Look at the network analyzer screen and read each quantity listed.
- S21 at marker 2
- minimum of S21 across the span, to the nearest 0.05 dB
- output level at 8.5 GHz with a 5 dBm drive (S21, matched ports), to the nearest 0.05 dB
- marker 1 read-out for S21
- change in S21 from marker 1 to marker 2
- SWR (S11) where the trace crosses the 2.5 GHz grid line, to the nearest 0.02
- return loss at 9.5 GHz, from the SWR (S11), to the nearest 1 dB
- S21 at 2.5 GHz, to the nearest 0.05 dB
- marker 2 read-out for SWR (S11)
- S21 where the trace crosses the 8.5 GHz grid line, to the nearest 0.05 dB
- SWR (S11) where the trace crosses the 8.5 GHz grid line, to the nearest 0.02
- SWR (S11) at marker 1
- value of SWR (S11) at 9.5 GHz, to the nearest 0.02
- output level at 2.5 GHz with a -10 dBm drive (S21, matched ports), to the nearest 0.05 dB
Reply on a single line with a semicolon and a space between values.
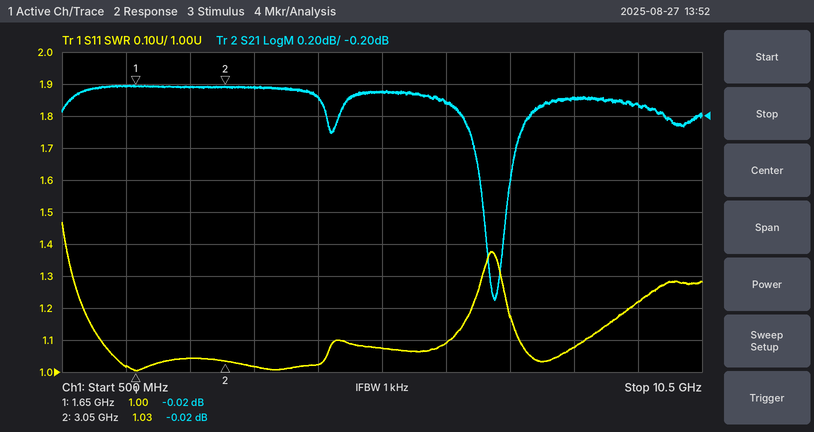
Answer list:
-0.02 dB; -1.35 dB; 4.90 dBm; -0.02 dB; 0.00 dB; 1.04; 20 dB; 0.00 dB; 1.03; -0.10 dB; 1.08; 1.00; 1.22; -10.00 dBm
